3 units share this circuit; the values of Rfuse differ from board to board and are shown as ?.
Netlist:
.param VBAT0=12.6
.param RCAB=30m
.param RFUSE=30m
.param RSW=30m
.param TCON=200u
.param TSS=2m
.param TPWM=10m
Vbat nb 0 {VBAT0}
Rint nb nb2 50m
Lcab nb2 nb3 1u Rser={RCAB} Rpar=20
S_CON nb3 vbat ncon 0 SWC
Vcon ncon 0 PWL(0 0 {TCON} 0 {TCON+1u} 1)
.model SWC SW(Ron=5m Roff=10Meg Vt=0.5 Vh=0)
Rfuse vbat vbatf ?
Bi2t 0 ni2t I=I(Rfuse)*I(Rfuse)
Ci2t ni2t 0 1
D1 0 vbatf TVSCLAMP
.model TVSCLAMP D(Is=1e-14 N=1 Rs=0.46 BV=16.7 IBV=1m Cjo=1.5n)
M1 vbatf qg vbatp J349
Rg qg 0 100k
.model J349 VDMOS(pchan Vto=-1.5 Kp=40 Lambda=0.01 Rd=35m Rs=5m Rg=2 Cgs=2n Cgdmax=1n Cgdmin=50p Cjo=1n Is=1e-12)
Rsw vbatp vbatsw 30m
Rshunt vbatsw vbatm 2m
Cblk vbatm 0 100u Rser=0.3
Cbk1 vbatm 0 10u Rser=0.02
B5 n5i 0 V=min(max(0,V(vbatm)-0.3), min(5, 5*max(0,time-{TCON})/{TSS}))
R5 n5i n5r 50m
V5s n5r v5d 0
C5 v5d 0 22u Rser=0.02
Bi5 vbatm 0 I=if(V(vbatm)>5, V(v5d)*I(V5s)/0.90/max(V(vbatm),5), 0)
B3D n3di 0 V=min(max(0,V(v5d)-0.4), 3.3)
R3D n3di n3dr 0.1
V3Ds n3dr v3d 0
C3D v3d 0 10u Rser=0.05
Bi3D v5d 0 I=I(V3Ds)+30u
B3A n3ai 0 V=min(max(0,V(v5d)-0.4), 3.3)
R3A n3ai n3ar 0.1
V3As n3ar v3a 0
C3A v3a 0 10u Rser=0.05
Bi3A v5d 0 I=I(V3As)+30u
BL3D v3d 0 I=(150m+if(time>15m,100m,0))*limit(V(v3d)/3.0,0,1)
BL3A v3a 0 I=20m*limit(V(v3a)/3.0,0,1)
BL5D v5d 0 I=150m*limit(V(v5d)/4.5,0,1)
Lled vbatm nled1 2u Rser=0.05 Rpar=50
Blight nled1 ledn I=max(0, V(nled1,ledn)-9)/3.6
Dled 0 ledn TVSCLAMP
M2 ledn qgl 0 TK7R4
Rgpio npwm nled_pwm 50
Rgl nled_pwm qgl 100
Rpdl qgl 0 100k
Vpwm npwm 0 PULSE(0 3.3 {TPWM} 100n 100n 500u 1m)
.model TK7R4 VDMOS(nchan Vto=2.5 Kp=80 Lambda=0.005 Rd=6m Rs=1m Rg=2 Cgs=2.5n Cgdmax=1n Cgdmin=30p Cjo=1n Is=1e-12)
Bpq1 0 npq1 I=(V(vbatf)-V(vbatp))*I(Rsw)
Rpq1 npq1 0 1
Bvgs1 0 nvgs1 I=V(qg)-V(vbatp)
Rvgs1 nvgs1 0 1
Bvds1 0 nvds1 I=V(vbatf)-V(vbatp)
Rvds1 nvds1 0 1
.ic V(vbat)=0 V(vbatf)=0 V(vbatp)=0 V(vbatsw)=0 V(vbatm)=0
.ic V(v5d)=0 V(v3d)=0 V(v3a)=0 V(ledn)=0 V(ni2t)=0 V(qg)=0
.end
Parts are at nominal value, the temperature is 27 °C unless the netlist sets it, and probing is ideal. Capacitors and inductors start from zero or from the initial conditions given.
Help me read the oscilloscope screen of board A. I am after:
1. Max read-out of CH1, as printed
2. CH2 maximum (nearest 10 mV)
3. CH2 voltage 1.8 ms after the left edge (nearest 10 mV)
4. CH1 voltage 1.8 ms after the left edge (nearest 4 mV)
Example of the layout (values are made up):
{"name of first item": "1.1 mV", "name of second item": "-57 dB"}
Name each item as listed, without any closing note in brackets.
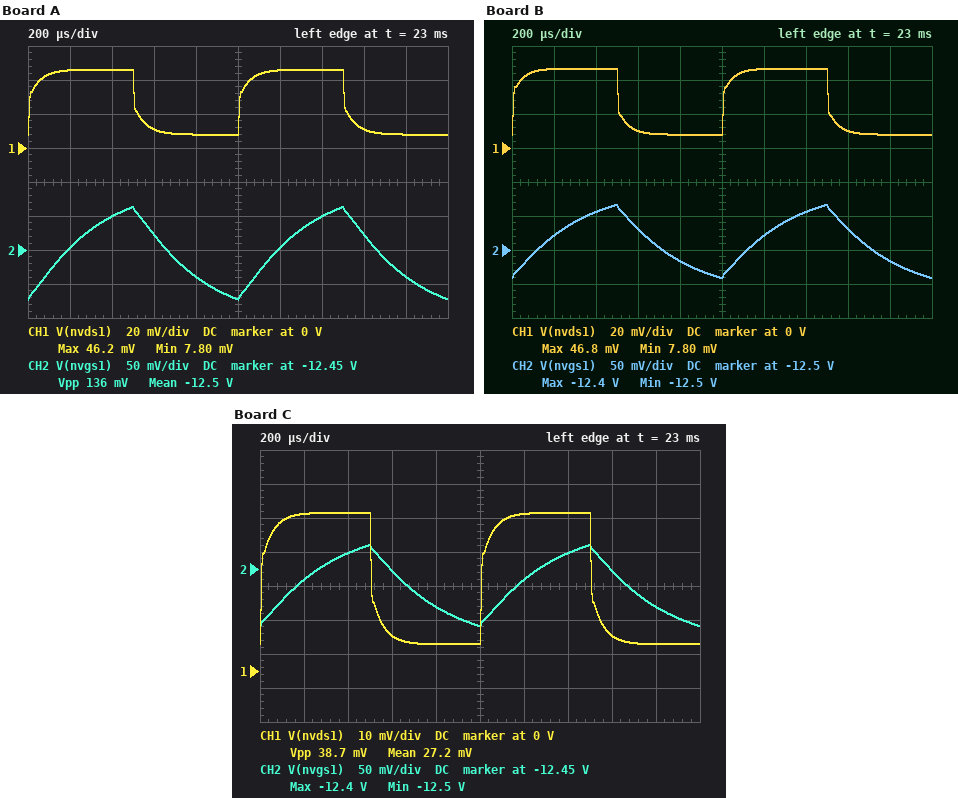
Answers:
{"Max read-out of CH1, as printed": "46.2 mV", "CH2 maximum": "-12.39 V", "CH2 voltage 1.8 ms after the left edge": "-12.49 V", "CH1 voltage 1.8 ms after the left edge": "8 mV"}
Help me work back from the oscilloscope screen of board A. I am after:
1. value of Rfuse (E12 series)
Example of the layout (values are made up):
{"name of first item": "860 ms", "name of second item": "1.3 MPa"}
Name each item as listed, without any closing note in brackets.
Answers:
{"value of Rfuse": "0.1 Ω"}
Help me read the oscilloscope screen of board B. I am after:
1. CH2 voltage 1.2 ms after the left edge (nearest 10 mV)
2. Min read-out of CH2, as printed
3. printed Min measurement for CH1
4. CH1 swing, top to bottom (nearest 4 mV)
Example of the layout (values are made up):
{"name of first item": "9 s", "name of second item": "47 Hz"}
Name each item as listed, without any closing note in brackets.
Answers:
{"CH2 voltage 1.2 ms after the left edge": "-12.48 V", "Min read-out of CH2, as printed": "-12.5 V", "printed Min measurement for CH1": "7.80 mV", "CH1 swing, top to bottom": "40 mV"}
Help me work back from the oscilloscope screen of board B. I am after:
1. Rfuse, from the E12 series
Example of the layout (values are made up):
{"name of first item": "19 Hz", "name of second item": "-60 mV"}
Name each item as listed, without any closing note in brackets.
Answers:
{"Rfuse, from the E12 series": "0.047 Ω"}
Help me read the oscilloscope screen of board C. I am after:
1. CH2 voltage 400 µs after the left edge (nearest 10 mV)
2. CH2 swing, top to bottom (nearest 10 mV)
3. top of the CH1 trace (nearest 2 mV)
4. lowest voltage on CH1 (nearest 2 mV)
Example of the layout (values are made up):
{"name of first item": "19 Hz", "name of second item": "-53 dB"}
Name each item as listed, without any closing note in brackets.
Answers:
{"CH2 voltage 400 µs after the left edge": "-12.43 V", "CH2 swing, top to bottom": "120 mV", "top of the CH1 trace": "46 mV", "lowest voltage on CH1": "8 mV"}
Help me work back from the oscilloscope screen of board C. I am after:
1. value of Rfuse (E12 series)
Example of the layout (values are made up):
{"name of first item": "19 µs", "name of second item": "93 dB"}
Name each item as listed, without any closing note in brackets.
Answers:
{"value of Rfuse": "0.068 Ω"}
